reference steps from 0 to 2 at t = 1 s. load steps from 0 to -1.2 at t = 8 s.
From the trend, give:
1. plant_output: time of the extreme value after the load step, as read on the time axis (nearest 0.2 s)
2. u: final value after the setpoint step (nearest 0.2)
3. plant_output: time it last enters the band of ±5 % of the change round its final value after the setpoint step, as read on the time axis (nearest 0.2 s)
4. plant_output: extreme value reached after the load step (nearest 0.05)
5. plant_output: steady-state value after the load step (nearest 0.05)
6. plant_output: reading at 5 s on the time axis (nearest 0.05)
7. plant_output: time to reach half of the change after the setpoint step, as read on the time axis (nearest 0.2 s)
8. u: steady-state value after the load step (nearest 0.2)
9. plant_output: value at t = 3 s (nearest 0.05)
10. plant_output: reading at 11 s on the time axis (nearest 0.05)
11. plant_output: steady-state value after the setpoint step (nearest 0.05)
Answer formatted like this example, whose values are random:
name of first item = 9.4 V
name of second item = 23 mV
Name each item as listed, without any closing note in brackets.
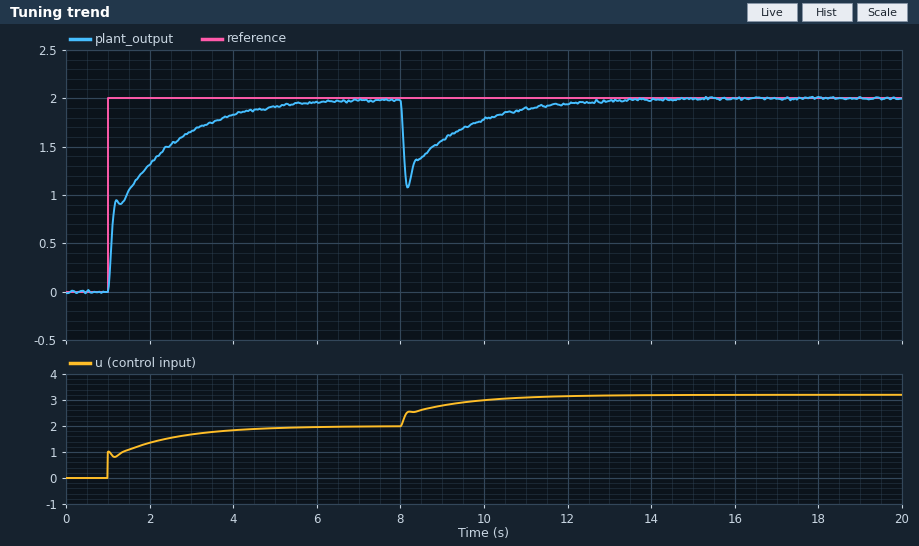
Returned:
plant_output: time of the extreme value after the load step, as read on the time axis = 8.2 s
u: final value after the setpoint step = 2.0
plant_output: time it last enters the band of ±5 % of the change round its final value after the setpoint step, as read on the time axis = 4.8 s
plant_output: extreme value reached after the load step = 1.10
plant_output: steady-state value after the load step = 2.00
plant_output: reading at 5 s on the time axis = 1.90
plant_output: time to reach half of the change after the setpoint step, as read on the time axis = 1.4 s
u: steady-state value after the load step = 3.2
plant_output: value at t = 3 s = 1.65
plant_output: reading at 11 s on the time axis = 1.90
plant_output: steady-state value after the setpoint step = 2.00
